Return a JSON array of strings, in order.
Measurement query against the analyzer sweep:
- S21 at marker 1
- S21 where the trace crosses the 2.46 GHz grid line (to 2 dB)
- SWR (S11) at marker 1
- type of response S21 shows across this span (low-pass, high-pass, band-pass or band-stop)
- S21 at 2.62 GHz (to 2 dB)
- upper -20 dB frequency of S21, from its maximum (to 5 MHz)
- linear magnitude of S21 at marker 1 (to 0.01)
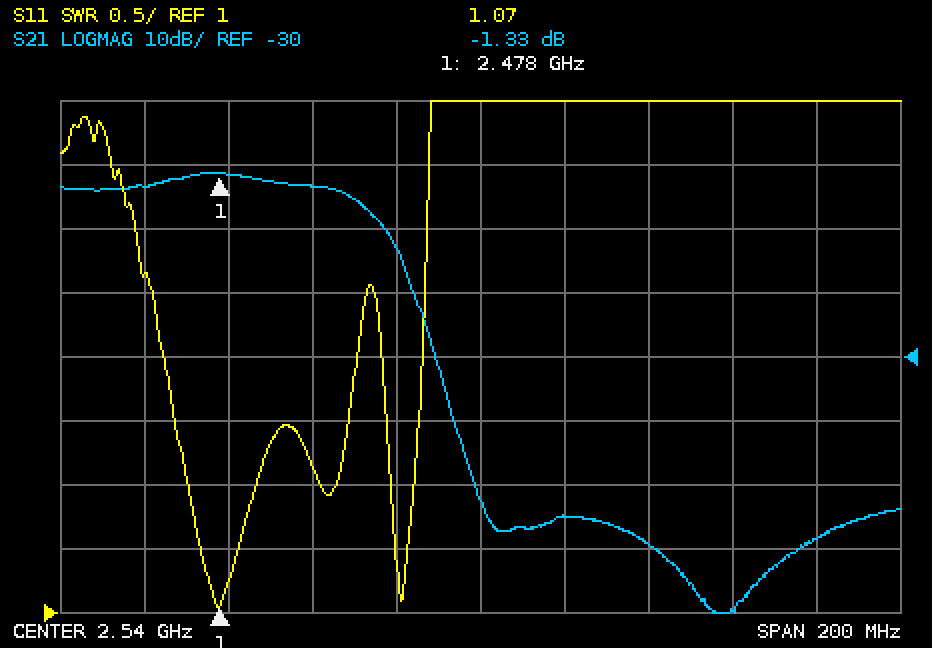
["-1.33 dB", "-4 dB", "1.07", "low-pass", "-58 dB", "2.525 GHz", "0.86"]
